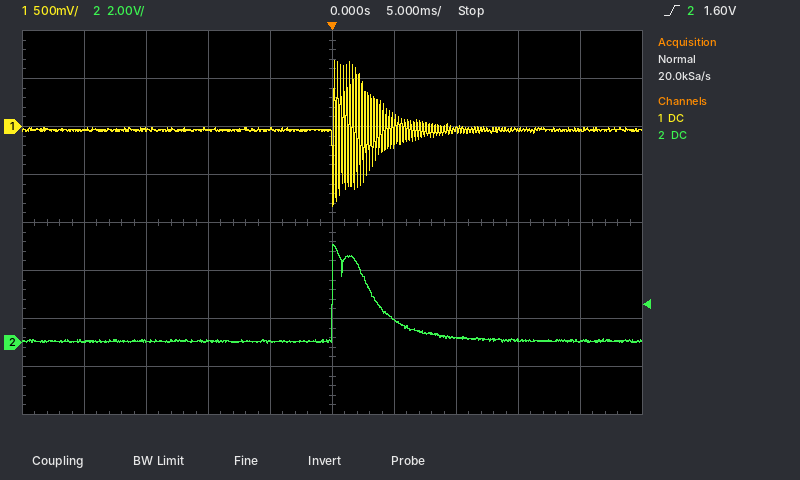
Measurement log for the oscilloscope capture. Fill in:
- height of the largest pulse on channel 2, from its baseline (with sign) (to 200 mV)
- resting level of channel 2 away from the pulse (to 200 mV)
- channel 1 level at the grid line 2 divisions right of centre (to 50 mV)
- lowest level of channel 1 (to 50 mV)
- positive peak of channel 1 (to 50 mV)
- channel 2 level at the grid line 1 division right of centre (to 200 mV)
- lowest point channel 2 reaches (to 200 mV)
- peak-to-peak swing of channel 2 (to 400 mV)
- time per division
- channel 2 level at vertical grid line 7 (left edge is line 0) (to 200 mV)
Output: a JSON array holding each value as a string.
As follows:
["+4.0 V", "0.0 V", "-50 mV", "-850 mV", "700 mV", "1.0 V", "0.0 V", "4.0 V", "5 ms", "200 mV"]
